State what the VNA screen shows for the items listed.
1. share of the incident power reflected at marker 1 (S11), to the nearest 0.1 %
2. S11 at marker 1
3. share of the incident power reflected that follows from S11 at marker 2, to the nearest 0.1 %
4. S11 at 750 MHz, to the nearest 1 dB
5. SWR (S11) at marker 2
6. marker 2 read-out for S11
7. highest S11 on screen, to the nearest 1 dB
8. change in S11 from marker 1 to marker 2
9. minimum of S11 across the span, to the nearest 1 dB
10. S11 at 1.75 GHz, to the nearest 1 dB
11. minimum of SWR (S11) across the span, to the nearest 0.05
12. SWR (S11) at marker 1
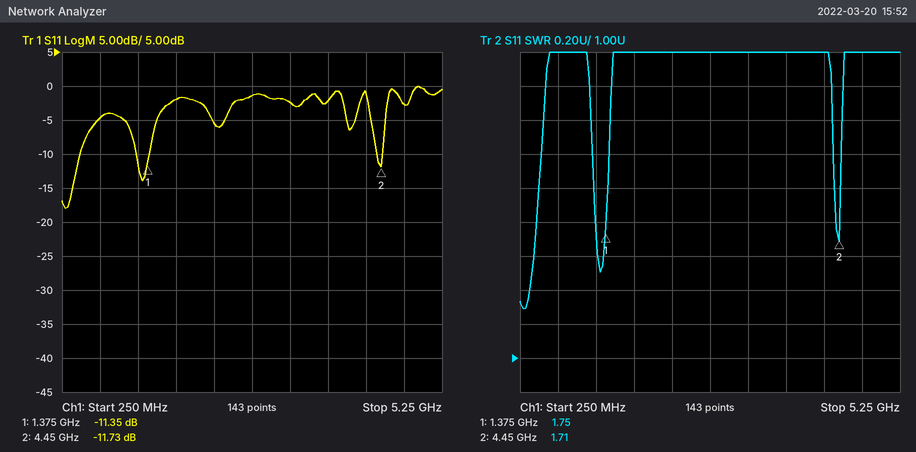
7.3 %
-11.35 dB
6.7 %
-5 dB
1.71
-11.73 dB
0 dB
-0.38 dB
-18 dB
-2 dB
1.30
1.75
